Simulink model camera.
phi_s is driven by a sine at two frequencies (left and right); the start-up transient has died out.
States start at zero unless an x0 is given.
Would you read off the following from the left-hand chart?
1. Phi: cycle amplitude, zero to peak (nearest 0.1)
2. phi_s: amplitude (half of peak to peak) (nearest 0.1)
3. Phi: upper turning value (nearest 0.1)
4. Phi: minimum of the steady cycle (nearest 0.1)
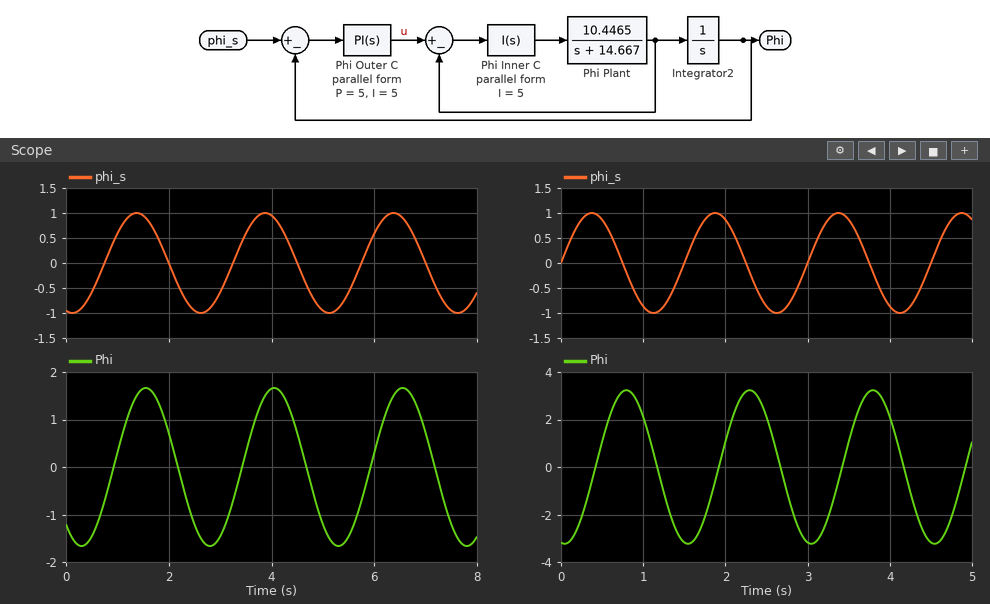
1.7
1.0
1.7
-1.7
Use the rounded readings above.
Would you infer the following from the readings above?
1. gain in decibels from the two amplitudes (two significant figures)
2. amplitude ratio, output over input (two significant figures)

4.6 dB
1.7
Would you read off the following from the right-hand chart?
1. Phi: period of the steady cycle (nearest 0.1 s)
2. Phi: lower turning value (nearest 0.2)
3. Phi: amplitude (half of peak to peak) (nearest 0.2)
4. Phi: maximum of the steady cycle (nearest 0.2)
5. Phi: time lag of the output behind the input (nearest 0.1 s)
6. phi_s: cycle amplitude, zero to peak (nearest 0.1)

1.5 s
-3.2
3.2
3.2
0.4 s
1.0
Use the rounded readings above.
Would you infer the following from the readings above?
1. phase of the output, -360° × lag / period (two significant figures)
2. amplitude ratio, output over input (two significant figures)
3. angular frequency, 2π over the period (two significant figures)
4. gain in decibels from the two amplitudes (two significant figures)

-96°
3.2
4.2 rad/s
10 dB
